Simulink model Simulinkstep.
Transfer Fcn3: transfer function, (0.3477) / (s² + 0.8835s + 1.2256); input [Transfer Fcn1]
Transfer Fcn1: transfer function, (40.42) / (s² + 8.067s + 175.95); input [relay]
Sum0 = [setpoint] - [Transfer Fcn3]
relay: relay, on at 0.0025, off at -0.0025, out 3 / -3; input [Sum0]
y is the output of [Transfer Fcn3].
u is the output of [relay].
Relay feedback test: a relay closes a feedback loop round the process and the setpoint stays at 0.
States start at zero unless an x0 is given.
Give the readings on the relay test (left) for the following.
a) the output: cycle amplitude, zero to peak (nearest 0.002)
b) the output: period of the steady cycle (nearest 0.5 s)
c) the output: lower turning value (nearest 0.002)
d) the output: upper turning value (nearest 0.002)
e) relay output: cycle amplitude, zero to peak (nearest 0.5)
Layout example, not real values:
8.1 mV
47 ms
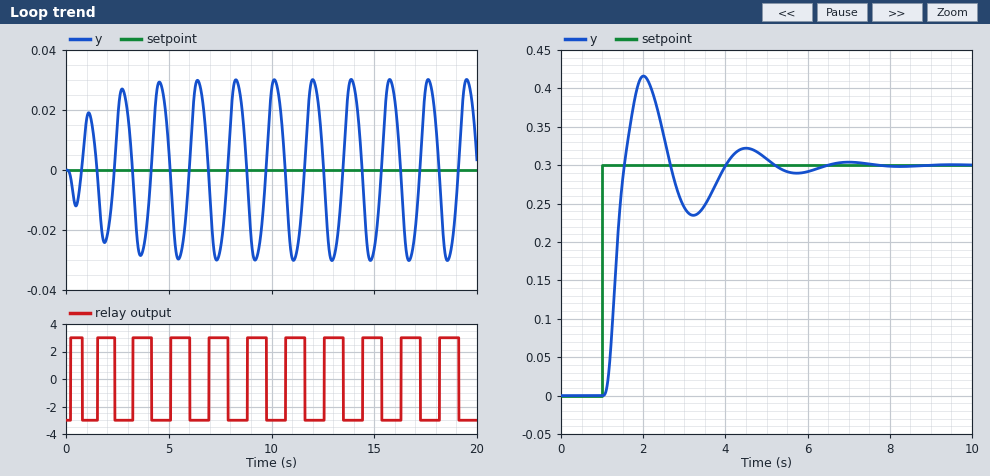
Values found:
0.030
2.0 s
-0.030
0.030
3.0
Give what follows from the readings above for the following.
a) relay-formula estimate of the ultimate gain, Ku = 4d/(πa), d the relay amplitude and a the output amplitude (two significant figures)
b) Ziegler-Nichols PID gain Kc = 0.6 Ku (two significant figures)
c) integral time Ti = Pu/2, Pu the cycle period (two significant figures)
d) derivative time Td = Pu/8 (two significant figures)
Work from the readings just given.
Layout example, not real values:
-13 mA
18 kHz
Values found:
130
78
1.0 s
0.25 s
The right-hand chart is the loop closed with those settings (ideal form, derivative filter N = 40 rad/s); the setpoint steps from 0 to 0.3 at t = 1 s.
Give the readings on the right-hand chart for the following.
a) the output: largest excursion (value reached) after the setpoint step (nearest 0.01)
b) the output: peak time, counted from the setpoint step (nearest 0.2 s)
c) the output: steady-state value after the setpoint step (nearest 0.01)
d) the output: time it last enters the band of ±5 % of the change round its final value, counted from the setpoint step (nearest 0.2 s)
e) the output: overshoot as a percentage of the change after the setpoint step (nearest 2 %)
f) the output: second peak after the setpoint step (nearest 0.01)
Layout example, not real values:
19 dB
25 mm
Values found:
0.42
1.0 s
0.30
3.8 s
38 %
0.32
